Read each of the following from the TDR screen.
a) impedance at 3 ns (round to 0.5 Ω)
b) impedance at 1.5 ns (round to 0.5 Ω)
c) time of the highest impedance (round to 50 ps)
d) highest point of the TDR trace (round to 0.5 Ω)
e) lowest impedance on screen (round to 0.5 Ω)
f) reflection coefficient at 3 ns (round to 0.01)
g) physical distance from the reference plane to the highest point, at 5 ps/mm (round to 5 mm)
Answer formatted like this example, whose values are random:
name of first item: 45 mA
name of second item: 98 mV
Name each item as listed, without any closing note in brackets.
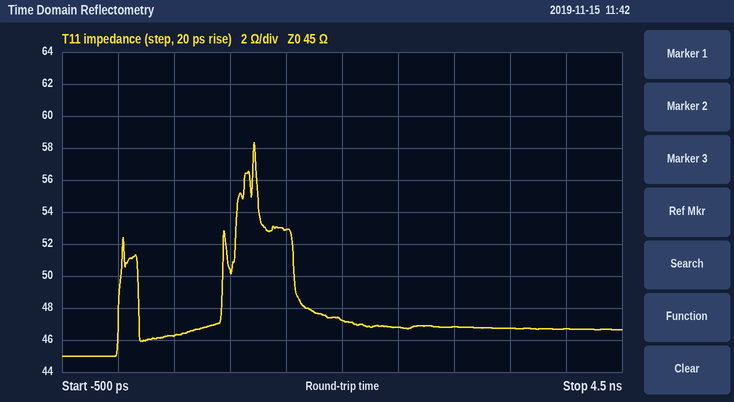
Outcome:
impedance at 3 ns: 47.0 Ω
impedance at 1.5 ns: 53.0 Ω
time of the highest impedance: 1.20 ns
highest point of the TDR trace: 58.5 Ω
lowest impedance on screen: 45.0 Ω
reflection coefficient at 3 ns: +0.02
physical distance from the reference plane to the highest point, at 5 ps/mm: 120 mm
